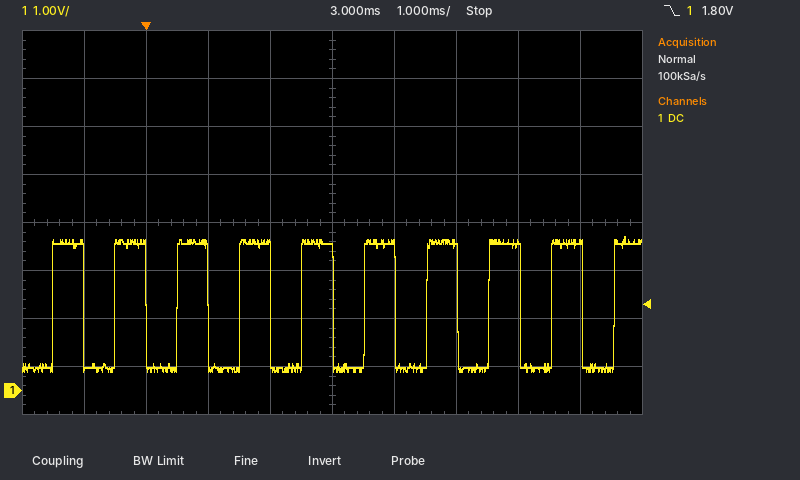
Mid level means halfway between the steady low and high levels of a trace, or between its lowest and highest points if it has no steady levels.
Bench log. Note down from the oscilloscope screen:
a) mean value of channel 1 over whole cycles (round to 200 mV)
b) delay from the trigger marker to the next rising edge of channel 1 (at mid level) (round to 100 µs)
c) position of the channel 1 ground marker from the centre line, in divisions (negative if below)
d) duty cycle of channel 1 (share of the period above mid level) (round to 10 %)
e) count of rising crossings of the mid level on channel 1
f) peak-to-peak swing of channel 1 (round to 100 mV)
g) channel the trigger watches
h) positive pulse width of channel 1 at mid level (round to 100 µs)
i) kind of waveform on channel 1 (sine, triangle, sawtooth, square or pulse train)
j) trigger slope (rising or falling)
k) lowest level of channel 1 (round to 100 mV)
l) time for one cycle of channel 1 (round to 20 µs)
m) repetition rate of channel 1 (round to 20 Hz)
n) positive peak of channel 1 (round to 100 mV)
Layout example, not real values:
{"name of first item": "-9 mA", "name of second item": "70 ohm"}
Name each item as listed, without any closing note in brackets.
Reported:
{"mean value of channel 1 over whole cycles": "1.8 V", "delay from the trigger marker to the next rising edge of channel 1 (at mid level)": "500 µs", "position of the channel 1 ground marker from the centre line, in divisions": "-3.5 div", "duty cycle of channel 1 (share of the period above mid level)": "50 %", "count of rising crossings of the mid level on channel 1": "10", "peak-to-peak swing of channel 1": "2.8 V", "channel the trigger watches": "channel 1", "positive pulse width of channel 1 at mid level": "500 µs", "kind of waveform on channel 1": "square", "trigger slope": "falling", "lowest level of channel 1": "400 mV", "time for one cycle of channel 1": "1.00 ms", "repetition rate of channel 1": "1.00 kHz", "positive peak of channel 1": "3.2 V"}
